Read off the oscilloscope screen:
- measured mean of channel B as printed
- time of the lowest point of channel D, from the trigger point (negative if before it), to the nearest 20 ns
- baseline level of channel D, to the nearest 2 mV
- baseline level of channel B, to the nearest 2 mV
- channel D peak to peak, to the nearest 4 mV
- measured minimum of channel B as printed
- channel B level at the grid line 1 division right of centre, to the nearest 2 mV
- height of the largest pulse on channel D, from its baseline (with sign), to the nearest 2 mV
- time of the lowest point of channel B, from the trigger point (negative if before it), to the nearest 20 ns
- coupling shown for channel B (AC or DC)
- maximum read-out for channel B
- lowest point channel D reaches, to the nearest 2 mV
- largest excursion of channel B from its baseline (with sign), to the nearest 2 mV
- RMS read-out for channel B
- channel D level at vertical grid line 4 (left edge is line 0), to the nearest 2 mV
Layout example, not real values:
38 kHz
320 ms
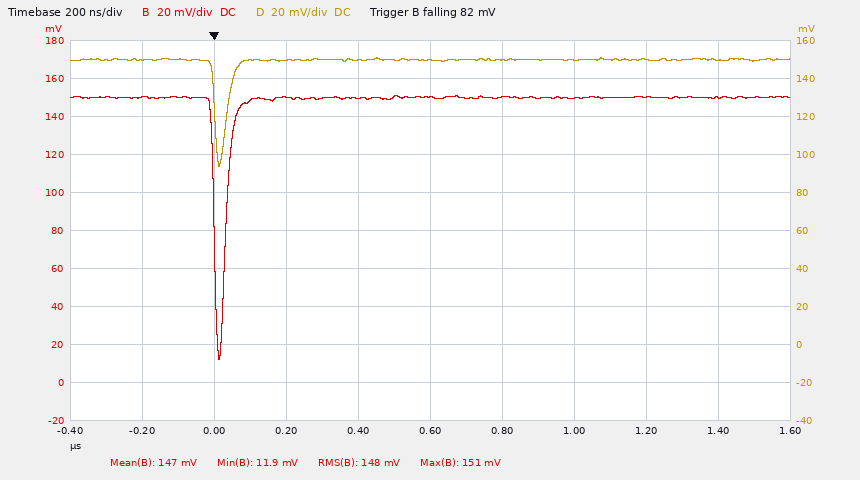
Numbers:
147 mV
+20 ns
150 mV
150 mV
56 mV
11.9 mV
150 mV
-56 mV
+20 ns
DC
151 mV
94 mV
-138 mV
148 mV
150 mV
